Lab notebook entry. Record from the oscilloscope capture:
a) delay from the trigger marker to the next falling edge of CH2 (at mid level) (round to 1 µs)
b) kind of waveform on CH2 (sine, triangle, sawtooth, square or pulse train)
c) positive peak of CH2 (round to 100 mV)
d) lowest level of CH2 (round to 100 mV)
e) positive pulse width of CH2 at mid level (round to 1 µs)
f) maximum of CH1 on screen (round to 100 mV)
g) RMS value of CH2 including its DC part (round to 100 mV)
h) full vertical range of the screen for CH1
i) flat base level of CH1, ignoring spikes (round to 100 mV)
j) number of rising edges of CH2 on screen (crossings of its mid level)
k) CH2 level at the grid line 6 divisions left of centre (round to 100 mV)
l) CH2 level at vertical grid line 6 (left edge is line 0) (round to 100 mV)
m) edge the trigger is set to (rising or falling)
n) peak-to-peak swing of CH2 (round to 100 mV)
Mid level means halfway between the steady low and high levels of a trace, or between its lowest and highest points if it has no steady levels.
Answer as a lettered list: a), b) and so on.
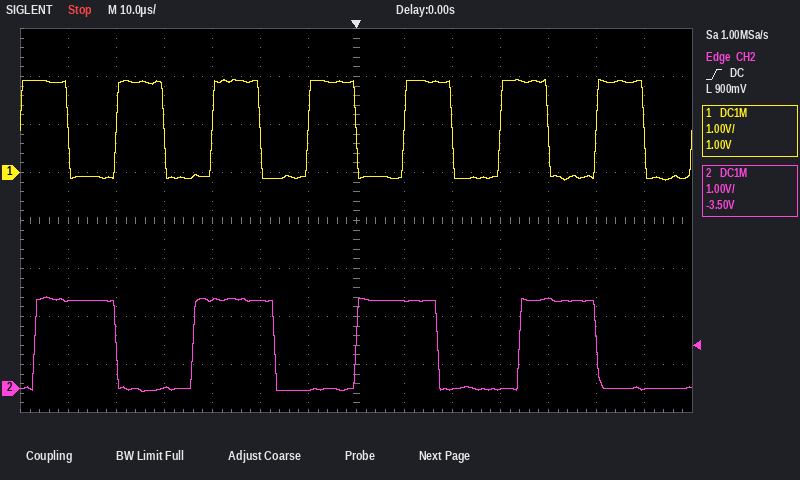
a) 17 µs
b) square
c) 1.9 V
d) -100 mV
e) 17 µs
f) 1.9 V
g) 1.3 V
h) 8 V
i) -100 mV
j) 4
k) 1.8 V
l) 0.0 V
m) rising
n) 2.0 V
